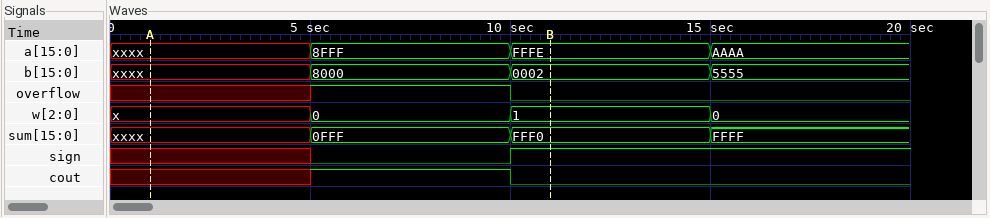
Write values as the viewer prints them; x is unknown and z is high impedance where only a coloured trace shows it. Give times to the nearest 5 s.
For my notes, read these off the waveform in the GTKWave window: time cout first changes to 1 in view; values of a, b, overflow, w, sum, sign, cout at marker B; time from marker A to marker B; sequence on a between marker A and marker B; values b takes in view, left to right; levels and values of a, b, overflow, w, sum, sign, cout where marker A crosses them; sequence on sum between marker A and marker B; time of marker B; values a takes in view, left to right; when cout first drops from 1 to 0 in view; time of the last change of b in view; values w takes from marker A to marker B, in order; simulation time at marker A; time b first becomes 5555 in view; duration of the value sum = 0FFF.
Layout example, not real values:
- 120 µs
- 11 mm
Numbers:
- 5 s
- a=FFFE, b=0002, overflow=0, w=1, sum=FFF0, sign=1, cout=0
- 10 s
- xxxx, 8FFF, FFFE
- xxxx, 8000, 0002, 5555
- a=xxxx, b=xxxx, overflow=x, w=x, sum=xxxx, sign=x, cout=x
- xxxx, 0FFF, FFF0
- 10 s
- xxxx, 8FFF, FFFE, AAAA
- 10 s
- 15 s
- x, 0, 1
- 0 s
- 15 s
- 5 s
